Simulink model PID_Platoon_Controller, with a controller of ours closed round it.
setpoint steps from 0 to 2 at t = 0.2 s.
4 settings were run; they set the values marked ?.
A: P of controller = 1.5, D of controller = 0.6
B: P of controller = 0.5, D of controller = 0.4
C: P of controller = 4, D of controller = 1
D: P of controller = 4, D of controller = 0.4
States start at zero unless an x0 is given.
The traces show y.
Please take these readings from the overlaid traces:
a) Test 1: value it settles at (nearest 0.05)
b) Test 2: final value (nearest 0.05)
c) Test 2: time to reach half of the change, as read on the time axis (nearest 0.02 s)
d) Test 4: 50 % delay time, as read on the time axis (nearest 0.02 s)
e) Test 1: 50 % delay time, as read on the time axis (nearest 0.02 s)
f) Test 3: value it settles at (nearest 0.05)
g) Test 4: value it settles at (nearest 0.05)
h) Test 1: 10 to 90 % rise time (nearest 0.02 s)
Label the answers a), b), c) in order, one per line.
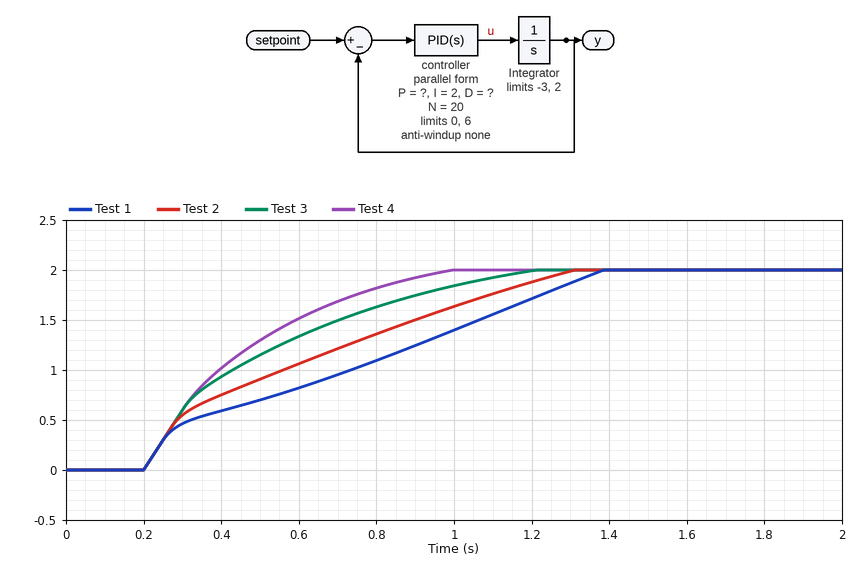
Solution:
a) 2.00
b) 2.00
c) 0.56 s
d) 0.40 s
e) 0.74 s
f) 2.00
g) 2.00
h) 1.02 s
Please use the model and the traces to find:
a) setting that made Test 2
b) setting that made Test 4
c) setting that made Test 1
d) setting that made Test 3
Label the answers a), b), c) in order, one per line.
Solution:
a) A
b) D
c) B
d) C
